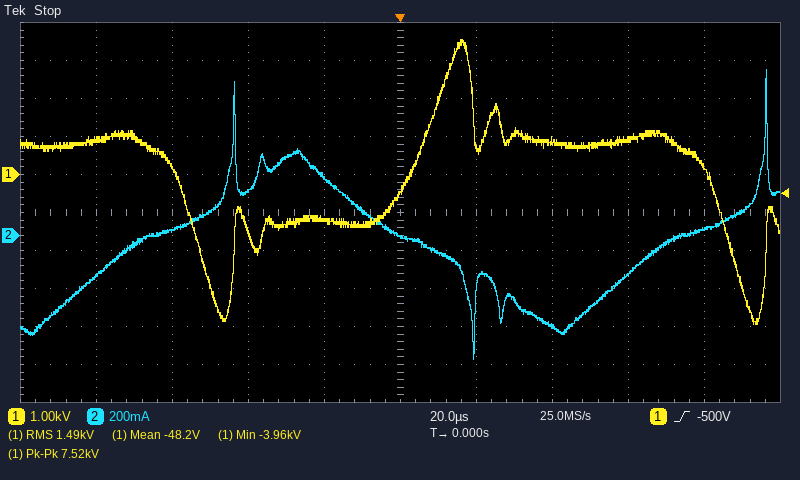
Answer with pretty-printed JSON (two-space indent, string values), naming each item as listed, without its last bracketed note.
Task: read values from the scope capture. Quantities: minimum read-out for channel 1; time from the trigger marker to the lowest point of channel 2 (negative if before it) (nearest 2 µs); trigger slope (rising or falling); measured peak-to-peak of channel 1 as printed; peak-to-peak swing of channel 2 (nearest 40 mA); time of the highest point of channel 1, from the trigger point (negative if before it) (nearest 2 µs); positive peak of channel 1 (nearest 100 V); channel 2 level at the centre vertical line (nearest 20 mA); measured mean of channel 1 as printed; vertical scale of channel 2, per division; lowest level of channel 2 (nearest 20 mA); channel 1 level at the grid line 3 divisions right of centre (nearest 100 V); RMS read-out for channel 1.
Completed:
{
  "minimum read-out for channel 1": "-3.96 kV",
  "time from the trigger marker to the lowest point of channel 2 (negative if before it)": "+20 µs",
  "trigger slope": "rising",
  "measured peak-to-peak of channel 1 as printed": "7.52 kV",
  "peak-to-peak swing of channel 2": "1.52 A",
  "time of the highest point of channel 1, from the trigger point (negative if before it)": "+16 µs",
  "positive peak of channel 1": "3.6 kV",
  "channel 2 level at the centre vertical line": "0 mA",
  "measured mean of channel 1 as printed": "-48.2 V",
  "vertical scale of channel 2, per division": "200 mA",
  "lowest level of channel 2": "-660 mA",
  "channel 1 level at the grid line 3 divisions right of centre": "900 V",
  "RMS read-out for channel 1": "1.49 kV"
}
